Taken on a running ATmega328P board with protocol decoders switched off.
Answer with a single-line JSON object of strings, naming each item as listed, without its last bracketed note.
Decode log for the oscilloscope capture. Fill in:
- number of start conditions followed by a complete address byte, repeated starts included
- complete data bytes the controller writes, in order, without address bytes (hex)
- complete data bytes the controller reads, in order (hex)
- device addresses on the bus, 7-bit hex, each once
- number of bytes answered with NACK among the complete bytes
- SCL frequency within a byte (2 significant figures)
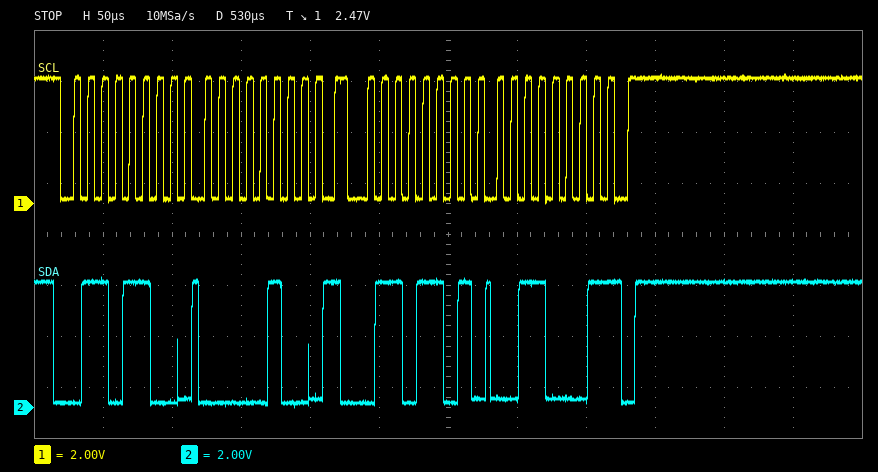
{"number of start conditions followed by a complete address byte, repeated starts included": "2", "complete data bytes the controller writes, in order, without address bytes": "04", "complete data bytes the controller reads, in order": "31", "device addresses on the bus, 7-bit hex, each once": "0x36", "number of bytes answered with NACK among the complete bytes": "1", "SCL frequency within a byte": "100 kHz"}
